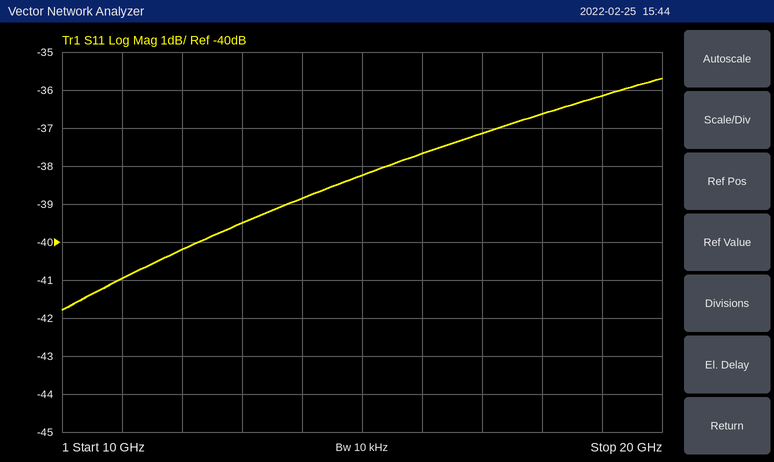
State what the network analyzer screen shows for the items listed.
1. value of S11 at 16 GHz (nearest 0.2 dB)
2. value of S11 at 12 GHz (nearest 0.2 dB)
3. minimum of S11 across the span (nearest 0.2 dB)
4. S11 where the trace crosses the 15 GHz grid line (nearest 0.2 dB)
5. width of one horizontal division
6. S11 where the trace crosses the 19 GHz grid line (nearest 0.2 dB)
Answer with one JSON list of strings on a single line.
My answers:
["-37.6 dB", "-40.2 dB", "-41.8 dB", "-38.2 dB", "1 GHz", "-36.2 dB"]
